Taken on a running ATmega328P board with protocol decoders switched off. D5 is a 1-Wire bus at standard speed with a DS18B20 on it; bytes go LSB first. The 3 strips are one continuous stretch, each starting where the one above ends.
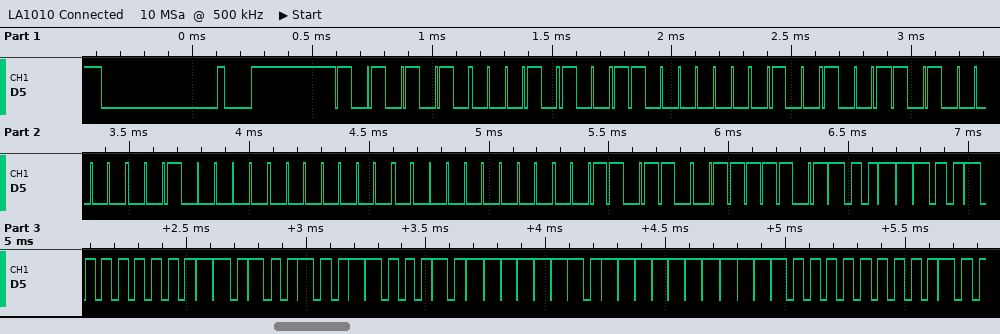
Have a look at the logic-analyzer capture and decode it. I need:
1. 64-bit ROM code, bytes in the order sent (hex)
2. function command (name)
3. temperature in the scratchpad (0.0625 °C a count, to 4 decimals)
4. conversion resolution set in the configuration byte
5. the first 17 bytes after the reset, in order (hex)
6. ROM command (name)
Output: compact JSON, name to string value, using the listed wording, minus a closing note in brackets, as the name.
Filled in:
{"64-bit ROM code, bytes in the order sent": "28 03 92 05 04 00 00 6C", "function command": "Read Scratchpad", "temperature in the scratchpad": "19.5625 °C", "conversion resolution set in the configuration byte": "12 bits", "the first 17 bytes after the reset, in order": "55 28 03 92 05 04 00 00 6C BE 39 01 4B 46 7F FF 07", "ROM command": "Match ROM"}
